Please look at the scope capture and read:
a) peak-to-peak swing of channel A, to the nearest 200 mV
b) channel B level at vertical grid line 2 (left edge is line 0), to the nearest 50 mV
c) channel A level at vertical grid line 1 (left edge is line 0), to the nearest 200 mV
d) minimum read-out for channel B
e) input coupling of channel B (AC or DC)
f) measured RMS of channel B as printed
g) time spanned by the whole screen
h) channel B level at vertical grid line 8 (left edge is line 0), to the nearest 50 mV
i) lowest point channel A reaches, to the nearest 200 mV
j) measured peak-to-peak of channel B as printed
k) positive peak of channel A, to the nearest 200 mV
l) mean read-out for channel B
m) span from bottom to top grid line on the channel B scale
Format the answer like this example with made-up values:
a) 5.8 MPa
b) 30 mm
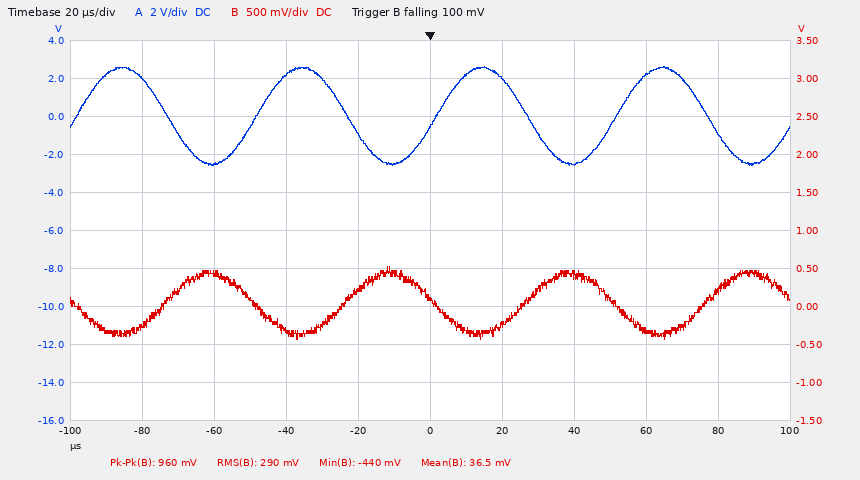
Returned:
a) 5.2 V
b) 450 mV
c) 2.0 V
d) -440 mV
e) DC
f) 290 mV
g) 200 µs
h) -300 mV
i) -2.6 V
j) 960 mV
k) 2.6 V
l) 36.5 mV
m) 5 V
